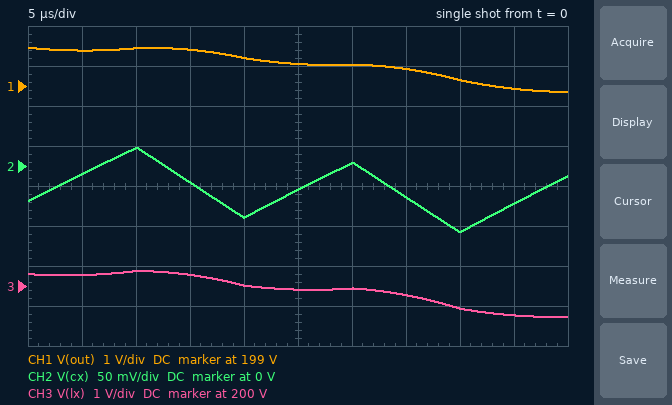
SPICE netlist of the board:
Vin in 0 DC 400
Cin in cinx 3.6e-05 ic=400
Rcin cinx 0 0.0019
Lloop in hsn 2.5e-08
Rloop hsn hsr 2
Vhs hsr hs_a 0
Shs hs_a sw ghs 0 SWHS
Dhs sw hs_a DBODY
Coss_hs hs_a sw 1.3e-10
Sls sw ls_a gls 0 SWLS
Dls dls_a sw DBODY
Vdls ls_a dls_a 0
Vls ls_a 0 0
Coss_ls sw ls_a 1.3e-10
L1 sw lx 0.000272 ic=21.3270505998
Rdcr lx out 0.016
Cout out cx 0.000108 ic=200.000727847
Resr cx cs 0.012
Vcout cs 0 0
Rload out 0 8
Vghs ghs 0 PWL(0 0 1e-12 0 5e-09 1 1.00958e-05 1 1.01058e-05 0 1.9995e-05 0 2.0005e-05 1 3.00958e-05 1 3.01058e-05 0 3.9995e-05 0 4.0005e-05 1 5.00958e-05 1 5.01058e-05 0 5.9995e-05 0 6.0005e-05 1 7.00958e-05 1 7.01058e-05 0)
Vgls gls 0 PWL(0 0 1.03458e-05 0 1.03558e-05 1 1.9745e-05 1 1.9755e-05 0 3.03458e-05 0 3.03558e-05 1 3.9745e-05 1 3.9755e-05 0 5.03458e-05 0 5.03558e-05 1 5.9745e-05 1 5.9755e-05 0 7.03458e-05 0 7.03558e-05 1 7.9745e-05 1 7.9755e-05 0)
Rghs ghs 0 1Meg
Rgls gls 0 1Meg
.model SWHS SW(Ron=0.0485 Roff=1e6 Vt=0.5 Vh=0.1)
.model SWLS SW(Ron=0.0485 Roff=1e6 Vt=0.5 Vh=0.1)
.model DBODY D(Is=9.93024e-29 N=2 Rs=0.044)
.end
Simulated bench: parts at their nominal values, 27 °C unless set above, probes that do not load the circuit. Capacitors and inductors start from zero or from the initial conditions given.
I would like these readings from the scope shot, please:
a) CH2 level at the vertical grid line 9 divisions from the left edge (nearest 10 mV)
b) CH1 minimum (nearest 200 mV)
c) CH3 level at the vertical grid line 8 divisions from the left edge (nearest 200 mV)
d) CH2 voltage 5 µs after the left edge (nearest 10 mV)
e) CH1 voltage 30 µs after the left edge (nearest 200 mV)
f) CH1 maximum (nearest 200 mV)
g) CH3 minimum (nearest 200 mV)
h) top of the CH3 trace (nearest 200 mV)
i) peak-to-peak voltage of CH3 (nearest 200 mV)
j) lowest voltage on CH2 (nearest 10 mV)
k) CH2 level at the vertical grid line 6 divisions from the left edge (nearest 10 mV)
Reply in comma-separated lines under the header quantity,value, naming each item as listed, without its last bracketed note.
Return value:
quantity,value
CH2 level at the vertical grid line 9 divisions from the left edge,-50 mV
CH1 minimum,198.8 V
CH3 level at the vertical grid line 8 divisions from the left edge,199.4 V
CH2 voltage 5 µs after the left edge,-10 mV
CH1 voltage 30 µs after the left edge,199.6 V
CH1 maximum,200.0 V
CH3 minimum,199.2 V
top of the CH3 trace,200.4 V
peak-to-peak voltage of CH3,1.2 V
lowest voltage on CH2,-80 mV
CH2 level at the vertical grid line 6 divisions from the left edge,0 V
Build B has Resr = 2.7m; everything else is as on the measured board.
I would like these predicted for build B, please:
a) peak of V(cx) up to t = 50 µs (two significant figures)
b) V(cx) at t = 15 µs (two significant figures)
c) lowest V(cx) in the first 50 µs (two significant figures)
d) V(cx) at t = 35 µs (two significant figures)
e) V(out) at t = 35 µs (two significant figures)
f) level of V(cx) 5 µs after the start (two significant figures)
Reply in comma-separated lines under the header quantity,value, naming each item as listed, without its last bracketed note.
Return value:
quantity,value
peak of V(cx) up to t = 50 µs,5.2 mV
V(cx) at t = 15 µs,-4.6 mV
lowest V(cx) in the first 50 µs,-19 mV
V(cx) at t = 35 µs,-8.8 mV
V(out) at t = 35 µs,200 V
level of V(cx) 5 µs after the start,-2.3 mV
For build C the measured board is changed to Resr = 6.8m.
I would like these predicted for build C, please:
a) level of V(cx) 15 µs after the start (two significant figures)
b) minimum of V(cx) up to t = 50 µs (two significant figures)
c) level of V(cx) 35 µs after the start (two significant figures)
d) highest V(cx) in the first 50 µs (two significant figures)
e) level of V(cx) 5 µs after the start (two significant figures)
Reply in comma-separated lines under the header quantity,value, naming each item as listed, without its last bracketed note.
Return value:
quantity,value
level of V(cx) 15 µs after the start,-12 mV
minimum of V(cx) up to t = 50 µs,-47 mV
level of V(cx) 35 µs after the start,-22 mV
highest V(cx) in the first 50 µs,13 mV
level of V(cx) 5 µs after the start,-5.8 mV
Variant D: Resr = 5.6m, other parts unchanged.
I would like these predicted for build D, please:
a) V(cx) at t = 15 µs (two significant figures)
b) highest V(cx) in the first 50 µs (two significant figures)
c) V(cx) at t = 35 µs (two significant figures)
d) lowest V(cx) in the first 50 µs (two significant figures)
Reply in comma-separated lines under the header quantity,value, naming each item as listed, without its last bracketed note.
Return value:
quantity,value
V(cx) at t = 15 µs,-9.6 mV
highest V(cx) in the first 50 µs,11 mV
V(cx) at t = 35 µs,-18 mV
lowest V(cx) in the first 50 µs,-39 mV
